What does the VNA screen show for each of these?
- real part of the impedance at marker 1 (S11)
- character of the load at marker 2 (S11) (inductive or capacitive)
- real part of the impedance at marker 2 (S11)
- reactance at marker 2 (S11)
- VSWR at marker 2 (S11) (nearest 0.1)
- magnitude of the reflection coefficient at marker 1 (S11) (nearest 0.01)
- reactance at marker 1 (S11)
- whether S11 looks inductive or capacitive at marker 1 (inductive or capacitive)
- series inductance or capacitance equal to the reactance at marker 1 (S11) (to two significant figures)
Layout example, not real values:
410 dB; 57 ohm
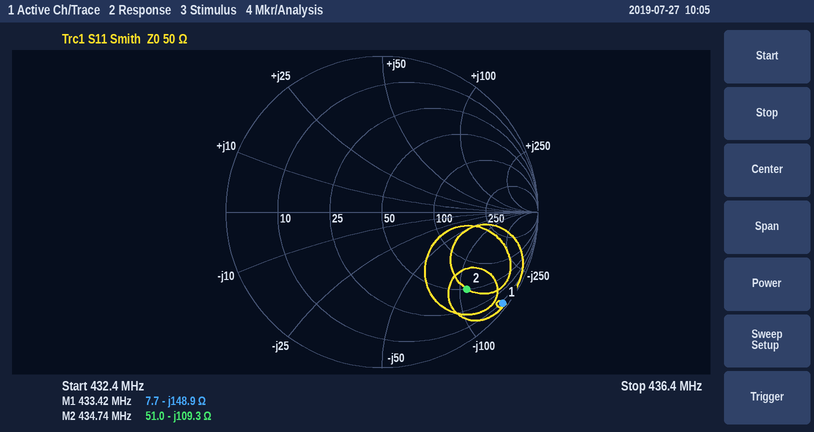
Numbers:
7.7 Ω; capacitive; 51.0 Ω; -109.3 Ω; 6.5; 0.97; -148.9 Ω; capacitive; 2.5 pF
